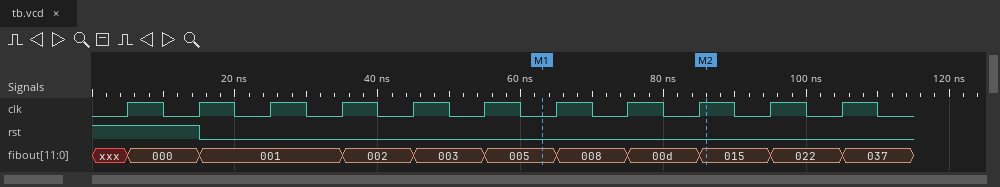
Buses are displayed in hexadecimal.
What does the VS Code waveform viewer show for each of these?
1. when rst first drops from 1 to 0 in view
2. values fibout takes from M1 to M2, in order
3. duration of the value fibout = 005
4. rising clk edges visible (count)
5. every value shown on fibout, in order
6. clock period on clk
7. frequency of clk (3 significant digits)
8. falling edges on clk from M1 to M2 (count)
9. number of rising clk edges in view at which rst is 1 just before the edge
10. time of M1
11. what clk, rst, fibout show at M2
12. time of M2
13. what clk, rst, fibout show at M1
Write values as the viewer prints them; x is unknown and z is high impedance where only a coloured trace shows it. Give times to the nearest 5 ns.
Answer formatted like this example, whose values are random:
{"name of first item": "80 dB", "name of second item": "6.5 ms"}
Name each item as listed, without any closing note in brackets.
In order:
{"when rst first drops from 1 to 0 in view": "15 ns", "values fibout takes from M1 to M2, in order": "005, 008, 00d, 015", "duration of the value fibout = 005": "10 ns", "rising clk edges visible": "11", "every value shown on fibout, in order": "xxx, 000, 001, 002, 003, 005, 008, 00d, 015, 022, 037", "clock period on clk": "10 ns", "frequency of clk": "100 MHz", "falling edges on clk from M1 to M2": "2", "number of rising clk edges in view at which rst is 1 just before the edge": "2", "time of M1": "65 ns", "what clk, rst, fibout show at M2": "clk=1, rst=0, fibout=015", "time of M2": "85 ns", "what clk, rst, fibout show at M1": "clk=0, rst=0, fibout=005"}
